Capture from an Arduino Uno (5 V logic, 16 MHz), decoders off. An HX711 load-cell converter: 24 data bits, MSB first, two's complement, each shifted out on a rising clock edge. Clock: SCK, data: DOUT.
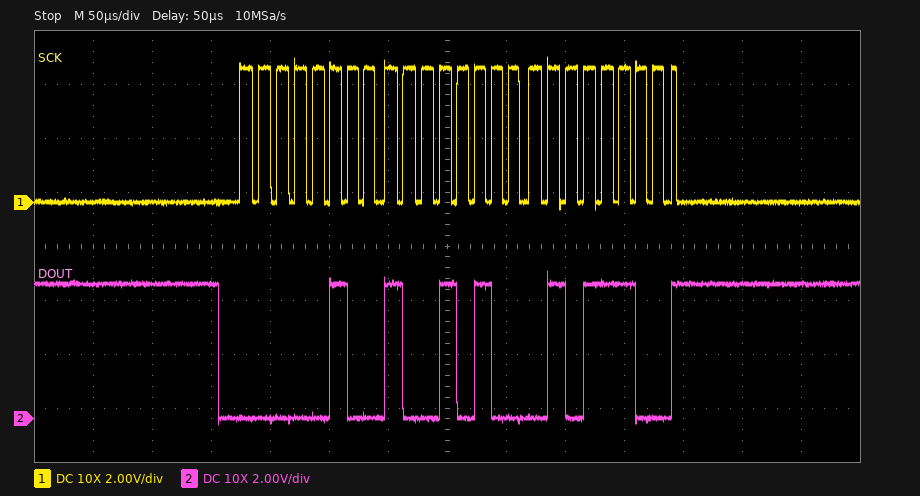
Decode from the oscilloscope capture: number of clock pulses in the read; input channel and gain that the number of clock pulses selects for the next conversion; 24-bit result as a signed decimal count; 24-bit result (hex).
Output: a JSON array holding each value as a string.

["25", "channel A, gain 128", "300124", "0x04945C"]
